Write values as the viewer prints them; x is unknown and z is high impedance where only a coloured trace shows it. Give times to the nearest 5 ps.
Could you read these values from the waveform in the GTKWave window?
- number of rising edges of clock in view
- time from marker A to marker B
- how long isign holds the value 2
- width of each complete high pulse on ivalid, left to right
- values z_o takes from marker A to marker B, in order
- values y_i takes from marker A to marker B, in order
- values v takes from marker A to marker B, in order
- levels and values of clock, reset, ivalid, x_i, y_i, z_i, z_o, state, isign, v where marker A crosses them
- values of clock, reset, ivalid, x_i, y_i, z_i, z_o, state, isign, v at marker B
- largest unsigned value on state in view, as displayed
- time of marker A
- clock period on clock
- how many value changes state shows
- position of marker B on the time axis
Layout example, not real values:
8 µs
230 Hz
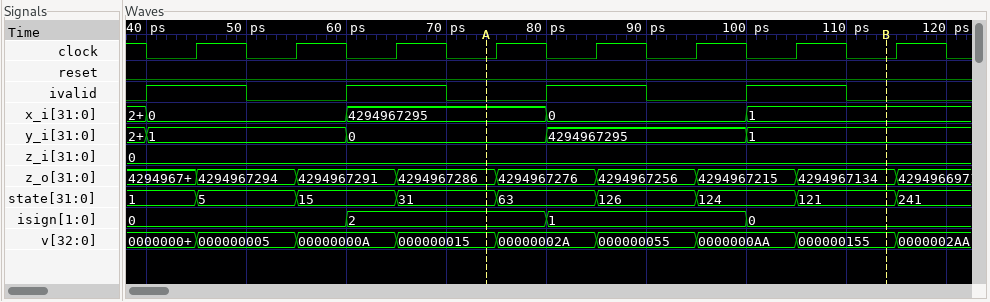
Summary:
8
40 ps
20 ps
10 ps, 10 ps, 10 ps, 10 ps
4294967286, 4294967276, 4294967256, 4294967215, 4294967134
0, 4294967295, 1
000000015, 00000002A, 000000055, 0000000AA, 000000155
clock=0, reset=0, ivalid=0, x_i=4294967295, y_i=0, z_i=0, z_o=4294967286, state=31, isign=2, v=000000015
clock=0, reset=0, ivalid=0, x_i=1, y_i=1, z_i=0, z_o=4294967134, state=121, isign=0, v=000000155
241
75 ps
10 ps
8
115 ps
